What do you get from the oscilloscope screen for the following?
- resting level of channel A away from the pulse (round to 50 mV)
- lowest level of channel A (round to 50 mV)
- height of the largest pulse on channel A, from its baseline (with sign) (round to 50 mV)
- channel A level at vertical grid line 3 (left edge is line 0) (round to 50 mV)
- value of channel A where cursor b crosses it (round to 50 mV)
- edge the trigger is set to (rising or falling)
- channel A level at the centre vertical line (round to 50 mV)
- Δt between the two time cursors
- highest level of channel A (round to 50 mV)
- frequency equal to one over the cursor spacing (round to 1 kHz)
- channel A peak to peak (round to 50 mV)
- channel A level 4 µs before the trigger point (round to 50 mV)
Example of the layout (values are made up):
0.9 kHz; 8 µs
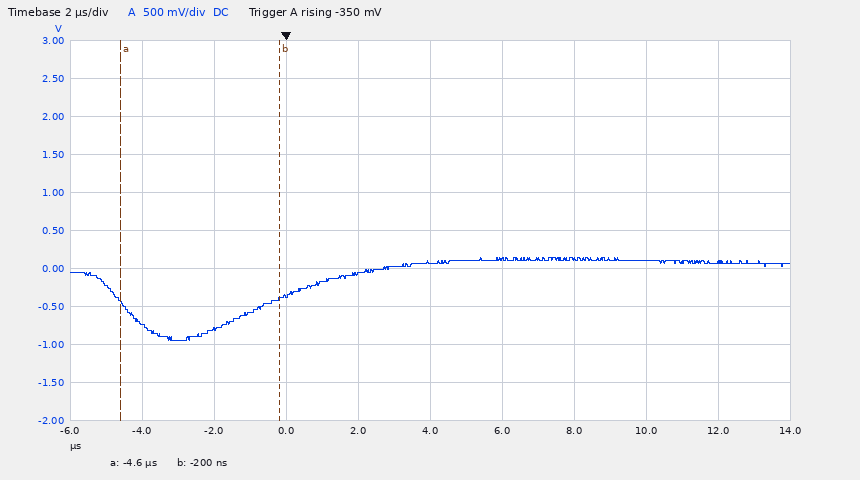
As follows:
100 mV; -950 mV; -1.05 V; -350 mV; -400 mV; rising; 100 mV; 4.4 µs; 150 mV; 227 kHz; 1.10 V; -750 mV
